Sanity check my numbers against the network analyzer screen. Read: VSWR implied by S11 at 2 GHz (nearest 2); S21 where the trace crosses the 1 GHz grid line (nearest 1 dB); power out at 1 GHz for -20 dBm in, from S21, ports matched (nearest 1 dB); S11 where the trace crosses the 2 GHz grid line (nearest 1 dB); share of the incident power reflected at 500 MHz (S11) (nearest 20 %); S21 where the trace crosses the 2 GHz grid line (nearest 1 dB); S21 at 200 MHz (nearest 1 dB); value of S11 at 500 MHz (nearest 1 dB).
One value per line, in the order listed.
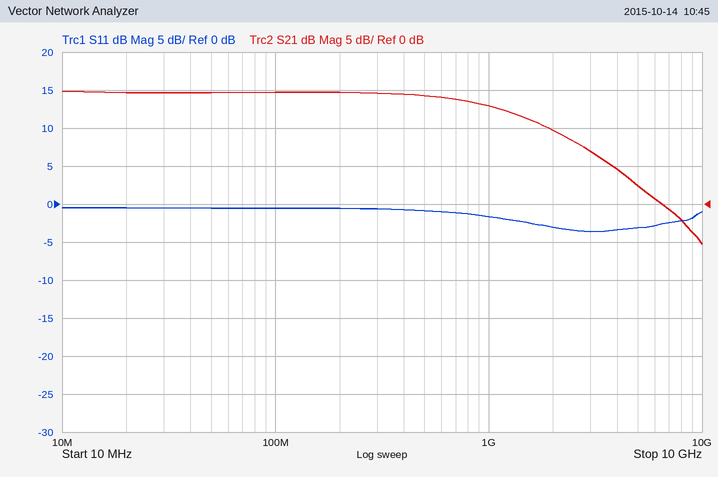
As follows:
6
13 dB
-7 dBm
-3 dB
80 %
10 dB
15 dB
-1 dB
